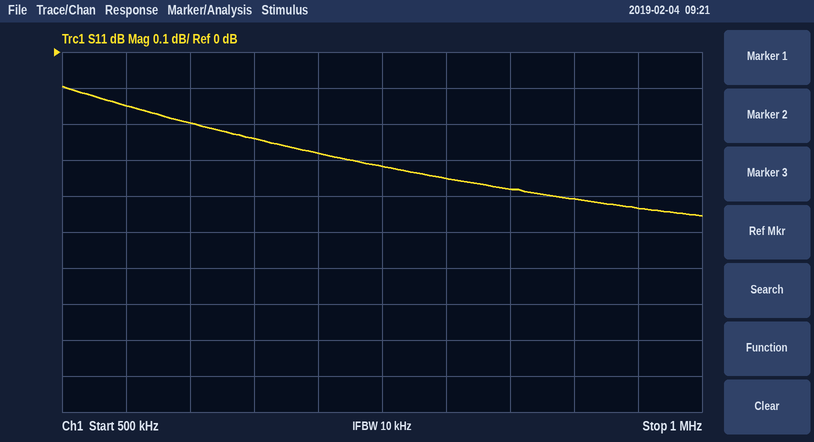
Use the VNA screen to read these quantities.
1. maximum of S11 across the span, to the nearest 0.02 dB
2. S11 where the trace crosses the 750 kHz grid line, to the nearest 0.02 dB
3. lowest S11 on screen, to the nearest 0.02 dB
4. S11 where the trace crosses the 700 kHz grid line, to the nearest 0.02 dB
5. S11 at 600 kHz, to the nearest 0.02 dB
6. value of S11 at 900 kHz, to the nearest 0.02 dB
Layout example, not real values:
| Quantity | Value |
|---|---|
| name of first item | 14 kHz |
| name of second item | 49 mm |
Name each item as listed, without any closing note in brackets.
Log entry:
| Quantity | Value |
|---|---|
| maximum of S11 across the span, to the nearest 0.02 dB | -0.10 dB |
| S11 where the trace crosses the 750 kHz grid line, to the nearest 0.02 dB | -0.32 dB |
| lowest S11 on screen, to the nearest 0.02 dB | -0.46 dB |
| S11 where the trace crosses the 700 kHz grid line, to the nearest 0.02 dB | -0.28 dB |
| S11 at 600 kHz, to the nearest 0.02 dB | -0.20 dB |
| value of S11 at 900 kHz, to the nearest 0.02 dB | -0.40 dB |
